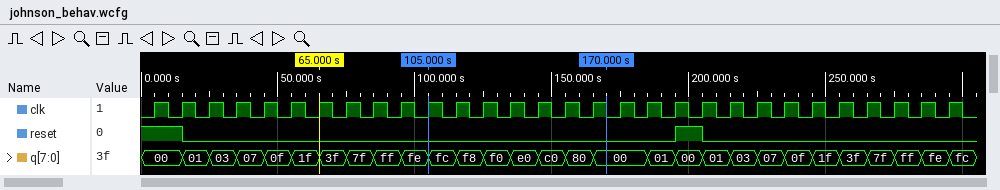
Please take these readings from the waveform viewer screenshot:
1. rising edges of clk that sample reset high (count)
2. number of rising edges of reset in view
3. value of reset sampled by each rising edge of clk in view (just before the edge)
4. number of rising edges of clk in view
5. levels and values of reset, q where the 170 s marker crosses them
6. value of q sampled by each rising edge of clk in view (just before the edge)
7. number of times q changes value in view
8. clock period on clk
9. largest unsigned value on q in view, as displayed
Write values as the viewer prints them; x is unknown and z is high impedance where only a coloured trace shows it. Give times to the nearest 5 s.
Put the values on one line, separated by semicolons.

3; 1; 1 1 0 0 0 0 0 0 0 0 0 0 0 0 0 0 0 0 0 0 1 0 0 0 0 0 0 0 0 0; 30; reset=0, q=00; 00, 00, 01, 03, 07, 0f, 1f, 3f, 7f, ff, fe, fc, f8, f0, e0, c0, 80, 00, 00, 01, 00, 01, 03, 07, 0f, 1f, 3f, 7f, ff, fe; 28; 10 s; ff
